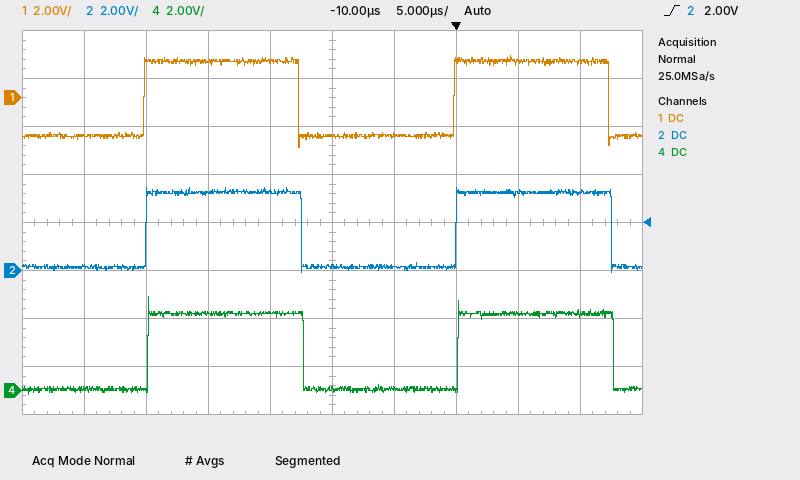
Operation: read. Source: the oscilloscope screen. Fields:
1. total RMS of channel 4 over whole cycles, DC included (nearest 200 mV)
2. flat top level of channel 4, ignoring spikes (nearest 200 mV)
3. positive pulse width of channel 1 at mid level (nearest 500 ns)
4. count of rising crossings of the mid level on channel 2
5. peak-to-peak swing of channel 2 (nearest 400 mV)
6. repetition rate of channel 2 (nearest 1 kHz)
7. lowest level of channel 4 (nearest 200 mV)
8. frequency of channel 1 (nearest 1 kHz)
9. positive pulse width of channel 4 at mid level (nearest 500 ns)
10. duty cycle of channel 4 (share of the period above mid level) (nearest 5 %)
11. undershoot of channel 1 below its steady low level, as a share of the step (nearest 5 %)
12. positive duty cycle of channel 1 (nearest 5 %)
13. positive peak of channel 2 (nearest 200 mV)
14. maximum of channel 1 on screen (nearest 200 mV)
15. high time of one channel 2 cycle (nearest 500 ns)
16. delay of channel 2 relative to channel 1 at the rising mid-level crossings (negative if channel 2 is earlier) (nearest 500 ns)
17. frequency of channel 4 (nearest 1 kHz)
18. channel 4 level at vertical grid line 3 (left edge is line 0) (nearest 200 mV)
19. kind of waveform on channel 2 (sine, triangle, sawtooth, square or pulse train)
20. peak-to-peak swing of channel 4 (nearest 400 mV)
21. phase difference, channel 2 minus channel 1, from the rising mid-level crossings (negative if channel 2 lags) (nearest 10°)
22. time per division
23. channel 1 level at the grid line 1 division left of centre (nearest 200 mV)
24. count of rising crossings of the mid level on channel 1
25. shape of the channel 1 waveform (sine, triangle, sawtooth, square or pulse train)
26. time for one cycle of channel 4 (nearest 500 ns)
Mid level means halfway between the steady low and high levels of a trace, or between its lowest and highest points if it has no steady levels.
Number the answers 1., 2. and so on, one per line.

1. 2.2 V
2. 3.2 V
3. 12.5 µs
4. 2
5. 3.6 V
6. 40 kHz
7. -200 mV
8. 40 kHz
9. 12.5 µs
10. 50 %
11. 15 %
12. 50 %
13. 3.4 V
14. 1.8 V
15. 12.5 µs
16. 0.0 µs
17. 40 kHz
18. 3.2 V
19. square
20. 4.0 V
21. 0°
22. 5 µs
23. 1.6 V
24. 2
25. square
26. 25.0 µs
